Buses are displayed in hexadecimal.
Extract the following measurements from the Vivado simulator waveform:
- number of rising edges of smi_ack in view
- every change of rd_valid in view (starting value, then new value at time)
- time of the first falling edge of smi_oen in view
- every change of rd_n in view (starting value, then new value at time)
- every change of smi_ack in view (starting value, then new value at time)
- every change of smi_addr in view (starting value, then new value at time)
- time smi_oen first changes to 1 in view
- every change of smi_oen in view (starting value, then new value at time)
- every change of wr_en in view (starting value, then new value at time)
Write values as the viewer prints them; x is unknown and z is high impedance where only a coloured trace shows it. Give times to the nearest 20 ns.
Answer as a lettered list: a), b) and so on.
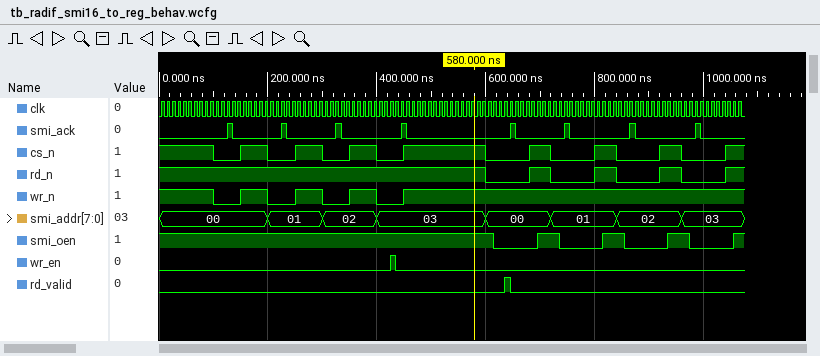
a) 8
b) 0, 1 at 640 ns, 0 at 640 ns
c) 620 ns
d) 1, 0 at 600 ns, 1 at 680 ns, 0 at 720 ns, 1 at 800 ns, 0 at 840 ns, 1 at 920 ns, 0 at 960 ns, 1 at 1040 ns
e) 0, 1 at 120 ns, 0 at 140 ns, 1 at 220 ns, 0 at 240 ns, 1 at 320 ns, 0 at 340 ns, 1 at 440 ns, 0 at 460 ns, 1 at 640 ns, 0 at 660 ns, 1 at 740 ns, 0 at 760 ns, 1 at 860 ns, 0 at 880 ns, 1 at 980 ns, 0 at 1000 ns
f) 00, 01 at 200 ns, 02 at 300 ns, 03 at 400 ns, 00 at 600 ns, 01 at 720 ns, 02 at 840 ns, 03 at 960 ns
g) 700 ns
h) 1, 0 at 620 ns, 1 at 700 ns, 0 at 740 ns, 1 at 820 ns, 0 at 860 ns, 1 at 940 ns, 0 at 980 ns, 1 at 1060 ns
i) 0, 1 at 420 ns, 0 at 440 ns
